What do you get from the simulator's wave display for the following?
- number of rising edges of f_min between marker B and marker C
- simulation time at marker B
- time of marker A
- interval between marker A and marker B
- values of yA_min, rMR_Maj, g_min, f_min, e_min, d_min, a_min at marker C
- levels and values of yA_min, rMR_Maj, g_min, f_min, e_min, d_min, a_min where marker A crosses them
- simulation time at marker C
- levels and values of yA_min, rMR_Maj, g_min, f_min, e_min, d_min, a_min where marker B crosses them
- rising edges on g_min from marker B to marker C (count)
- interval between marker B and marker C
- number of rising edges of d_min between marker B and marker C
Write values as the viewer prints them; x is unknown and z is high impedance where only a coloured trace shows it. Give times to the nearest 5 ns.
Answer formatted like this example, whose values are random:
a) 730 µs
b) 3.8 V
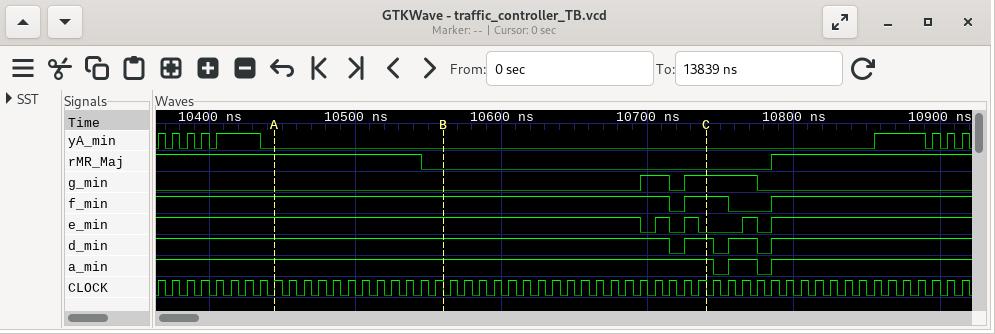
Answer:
a) 1
b) 10560 ns
c) 10445 ns
d) 115 ns
e) yA_min=0, rMR_Maj=0, g_min=1, f_min=1, e_min=0, d_min=1, a_min=1
f) yA_min=0, rMR_Maj=1, g_min=0, f_min=1, e_min=1, d_min=1, a_min=1
g) 10740 ns
h) yA_min=0, rMR_Maj=0, g_min=0, f_min=1, e_min=1, d_min=1, a_min=1
i) 2
j) 180 ns
k) 1
